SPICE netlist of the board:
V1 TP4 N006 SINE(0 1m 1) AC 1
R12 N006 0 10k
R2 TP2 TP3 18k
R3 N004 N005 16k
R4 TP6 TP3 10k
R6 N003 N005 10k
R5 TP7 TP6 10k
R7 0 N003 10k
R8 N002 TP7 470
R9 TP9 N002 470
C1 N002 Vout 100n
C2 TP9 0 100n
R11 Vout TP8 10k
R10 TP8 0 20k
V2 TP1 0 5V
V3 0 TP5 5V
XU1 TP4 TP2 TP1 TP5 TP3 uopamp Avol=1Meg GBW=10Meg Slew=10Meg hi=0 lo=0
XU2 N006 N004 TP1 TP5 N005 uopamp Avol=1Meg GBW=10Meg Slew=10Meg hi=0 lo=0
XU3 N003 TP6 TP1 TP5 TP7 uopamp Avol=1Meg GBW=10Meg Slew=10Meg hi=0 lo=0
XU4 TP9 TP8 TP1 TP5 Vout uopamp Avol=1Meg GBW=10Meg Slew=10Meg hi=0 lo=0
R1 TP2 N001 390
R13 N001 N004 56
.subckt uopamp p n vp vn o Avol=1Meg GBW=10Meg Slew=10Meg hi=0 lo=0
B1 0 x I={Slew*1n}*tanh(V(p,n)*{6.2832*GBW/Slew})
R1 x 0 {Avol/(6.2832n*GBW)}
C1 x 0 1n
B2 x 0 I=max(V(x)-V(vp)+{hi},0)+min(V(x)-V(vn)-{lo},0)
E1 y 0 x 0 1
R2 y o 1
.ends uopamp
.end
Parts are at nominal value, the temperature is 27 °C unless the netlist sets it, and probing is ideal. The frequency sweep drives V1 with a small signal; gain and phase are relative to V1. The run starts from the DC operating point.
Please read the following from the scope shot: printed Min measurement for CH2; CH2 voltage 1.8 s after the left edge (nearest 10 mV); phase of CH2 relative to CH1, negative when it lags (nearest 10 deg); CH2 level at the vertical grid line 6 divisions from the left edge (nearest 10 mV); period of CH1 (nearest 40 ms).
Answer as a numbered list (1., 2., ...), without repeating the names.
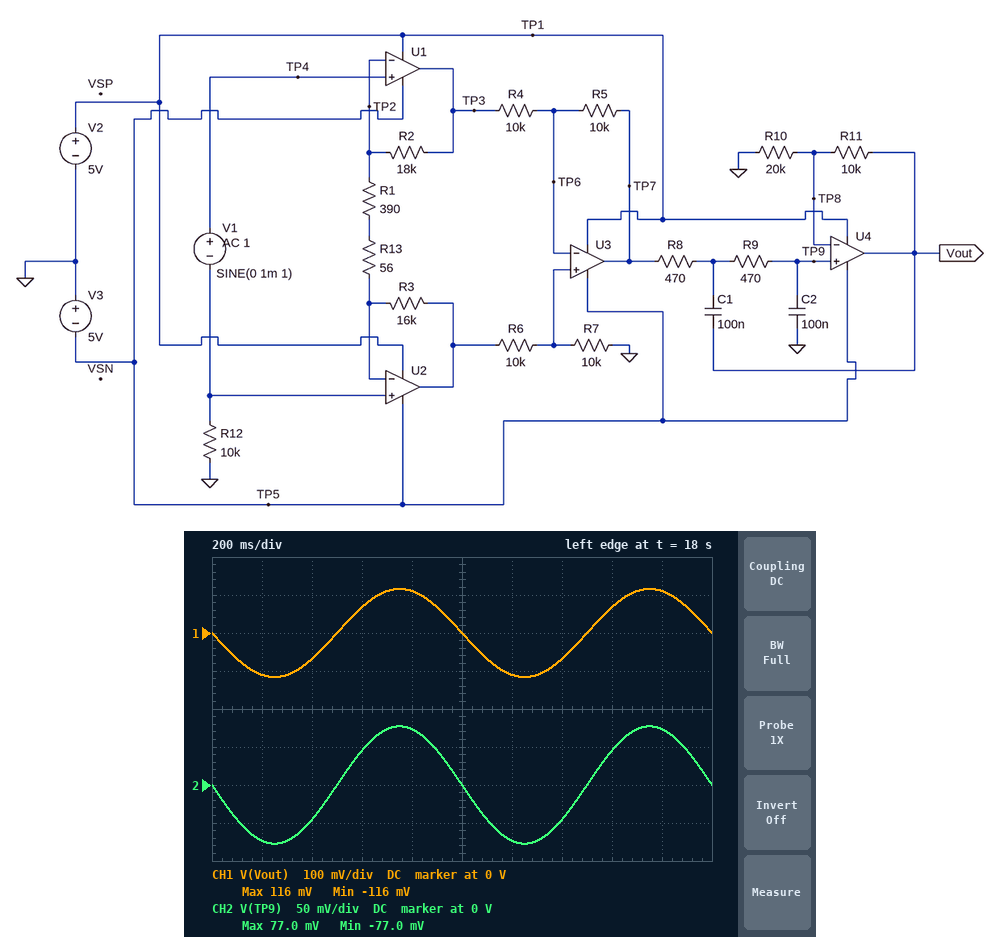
1. -77.0 mV
2. 70 mV
3. 0 deg
4. -70 mV
5. 1.00 s
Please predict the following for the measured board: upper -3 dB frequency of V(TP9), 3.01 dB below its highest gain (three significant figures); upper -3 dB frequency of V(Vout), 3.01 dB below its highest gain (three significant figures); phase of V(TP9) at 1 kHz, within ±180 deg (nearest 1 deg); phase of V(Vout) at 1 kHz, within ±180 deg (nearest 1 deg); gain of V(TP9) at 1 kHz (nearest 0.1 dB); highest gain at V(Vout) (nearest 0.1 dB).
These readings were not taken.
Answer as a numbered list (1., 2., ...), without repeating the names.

1. 3.18 kHz
2. 3.18 kHz
3. 154 deg
4. 154 deg
5. 37.6 dB
6. 41.3 dB
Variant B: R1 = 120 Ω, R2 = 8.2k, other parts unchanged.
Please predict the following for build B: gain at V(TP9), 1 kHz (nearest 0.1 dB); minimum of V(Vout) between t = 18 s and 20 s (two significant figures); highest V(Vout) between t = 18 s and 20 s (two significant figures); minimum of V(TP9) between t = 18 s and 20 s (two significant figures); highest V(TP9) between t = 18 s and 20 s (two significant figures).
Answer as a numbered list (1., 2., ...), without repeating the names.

1. 42.7 dB
2. -210 mV
3. 210 mV
4. -140 mV
5. 140 mV
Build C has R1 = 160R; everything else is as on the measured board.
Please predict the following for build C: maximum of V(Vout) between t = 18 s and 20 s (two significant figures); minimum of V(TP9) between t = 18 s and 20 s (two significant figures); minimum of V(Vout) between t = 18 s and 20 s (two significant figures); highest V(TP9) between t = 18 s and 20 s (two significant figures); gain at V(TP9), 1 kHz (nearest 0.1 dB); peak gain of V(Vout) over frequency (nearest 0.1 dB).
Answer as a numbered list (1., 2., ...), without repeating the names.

1. 240 mV
2. -160 mV
3. -240 mV
4. 160 mV
5. 43.9 dB
6. 47.5 dB
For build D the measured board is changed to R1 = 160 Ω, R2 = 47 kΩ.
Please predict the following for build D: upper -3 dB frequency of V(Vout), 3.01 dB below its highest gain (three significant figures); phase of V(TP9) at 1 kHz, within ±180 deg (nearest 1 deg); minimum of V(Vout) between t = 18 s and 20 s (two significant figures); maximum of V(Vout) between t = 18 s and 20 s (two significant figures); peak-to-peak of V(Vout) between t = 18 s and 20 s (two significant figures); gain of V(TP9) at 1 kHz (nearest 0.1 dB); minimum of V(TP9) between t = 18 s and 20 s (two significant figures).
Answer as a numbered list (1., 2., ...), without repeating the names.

1. 3.17 kHz
2. 152 deg
3. -440 mV
4. 440 mV
5. 880 mV
6. 49.2 dB
7. -290 mV
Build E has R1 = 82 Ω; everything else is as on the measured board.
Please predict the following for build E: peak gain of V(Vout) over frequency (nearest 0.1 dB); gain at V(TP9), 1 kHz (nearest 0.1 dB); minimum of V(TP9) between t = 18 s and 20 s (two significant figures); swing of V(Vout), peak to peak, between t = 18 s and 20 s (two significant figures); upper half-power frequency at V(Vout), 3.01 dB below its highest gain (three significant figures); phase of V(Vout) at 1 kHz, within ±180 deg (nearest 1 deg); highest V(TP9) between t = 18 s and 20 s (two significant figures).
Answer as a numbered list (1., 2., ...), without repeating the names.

1. 51.4 dB
2. 47.7 dB
3. -250 mV
4. 740 mV
5. 3.17 kHz
6. 153 deg
7. 250 mV
